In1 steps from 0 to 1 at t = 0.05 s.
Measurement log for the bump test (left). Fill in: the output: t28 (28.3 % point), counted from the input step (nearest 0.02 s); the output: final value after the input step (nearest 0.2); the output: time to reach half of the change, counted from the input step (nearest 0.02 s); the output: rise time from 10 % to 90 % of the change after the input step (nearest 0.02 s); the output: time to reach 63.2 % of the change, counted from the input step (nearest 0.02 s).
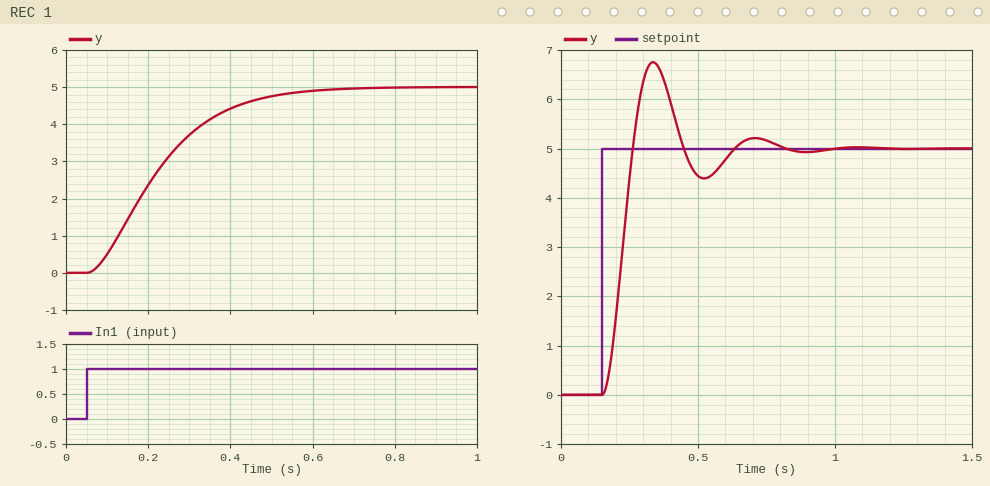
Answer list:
0.10 s
5.0
0.16 s
0.32 s
0.20 s
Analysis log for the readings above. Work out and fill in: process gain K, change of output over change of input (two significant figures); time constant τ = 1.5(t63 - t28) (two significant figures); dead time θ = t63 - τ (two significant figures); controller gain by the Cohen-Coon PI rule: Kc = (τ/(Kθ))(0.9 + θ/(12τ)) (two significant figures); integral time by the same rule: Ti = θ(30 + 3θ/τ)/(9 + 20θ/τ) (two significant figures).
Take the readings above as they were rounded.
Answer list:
5.0
0.15 s
0.050 s
0.56
0.099 s
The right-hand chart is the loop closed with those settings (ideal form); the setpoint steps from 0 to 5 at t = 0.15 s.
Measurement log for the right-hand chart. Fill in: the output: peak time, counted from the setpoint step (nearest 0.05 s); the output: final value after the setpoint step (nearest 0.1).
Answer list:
0.20 s
5.0
